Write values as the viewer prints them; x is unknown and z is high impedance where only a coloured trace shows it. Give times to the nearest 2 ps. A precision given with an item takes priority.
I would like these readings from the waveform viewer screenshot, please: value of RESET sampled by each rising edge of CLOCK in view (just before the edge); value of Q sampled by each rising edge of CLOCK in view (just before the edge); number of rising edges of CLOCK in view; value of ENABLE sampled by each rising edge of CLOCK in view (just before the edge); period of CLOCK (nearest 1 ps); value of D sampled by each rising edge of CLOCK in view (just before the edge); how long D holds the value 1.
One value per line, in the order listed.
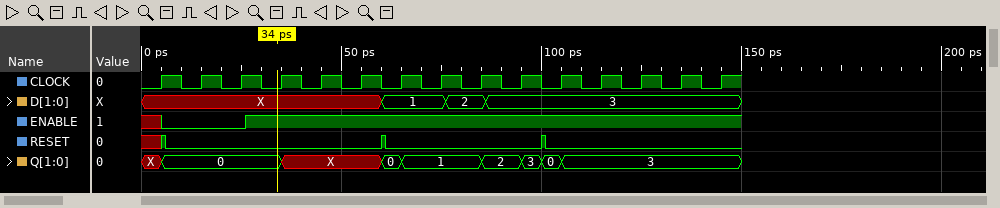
x 0 0 0 0 0 0 0 0 0 0 0 0 0 0
X, 0, 0, 0, X, X, 0, 1, 1, 2, 0, 3, 3, 3, 3
15
x 0 0 1 1 1 1 1 1 1 1 1 1 1 1
10 ps
X, X, X, X, X, X, 1, 1, 2, 3, 3, 3, 3, 3, 3
16 ps
